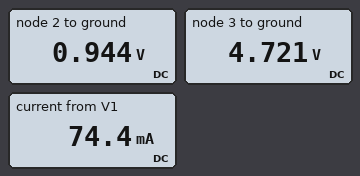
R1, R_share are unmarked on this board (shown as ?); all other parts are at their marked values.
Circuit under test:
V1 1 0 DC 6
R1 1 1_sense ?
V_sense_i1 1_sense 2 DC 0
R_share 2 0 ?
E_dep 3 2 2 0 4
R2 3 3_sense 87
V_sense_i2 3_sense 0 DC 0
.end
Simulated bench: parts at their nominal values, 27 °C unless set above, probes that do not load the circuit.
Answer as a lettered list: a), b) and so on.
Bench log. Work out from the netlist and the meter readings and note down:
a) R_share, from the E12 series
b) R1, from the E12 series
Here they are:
a) 47 Ω
b) 68 Ω
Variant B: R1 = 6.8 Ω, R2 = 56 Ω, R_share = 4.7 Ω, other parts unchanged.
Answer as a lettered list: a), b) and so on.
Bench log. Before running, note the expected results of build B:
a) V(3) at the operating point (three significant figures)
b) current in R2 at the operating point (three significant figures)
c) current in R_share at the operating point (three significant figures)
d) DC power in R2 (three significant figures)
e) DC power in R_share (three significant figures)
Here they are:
a) 9.82 V
b) 175 mA
c) 418 mA
d) 1.72 W
e) 821 mW
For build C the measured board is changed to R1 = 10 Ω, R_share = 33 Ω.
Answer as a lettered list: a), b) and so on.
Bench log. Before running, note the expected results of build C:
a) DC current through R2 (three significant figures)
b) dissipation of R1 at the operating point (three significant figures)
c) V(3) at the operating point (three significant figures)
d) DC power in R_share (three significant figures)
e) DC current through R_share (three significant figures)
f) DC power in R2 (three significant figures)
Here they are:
a) 184 mA
b) 787 mW
c) 16.0 V
d) 309 mW
e) 96.8 mA
f) 2.93 W
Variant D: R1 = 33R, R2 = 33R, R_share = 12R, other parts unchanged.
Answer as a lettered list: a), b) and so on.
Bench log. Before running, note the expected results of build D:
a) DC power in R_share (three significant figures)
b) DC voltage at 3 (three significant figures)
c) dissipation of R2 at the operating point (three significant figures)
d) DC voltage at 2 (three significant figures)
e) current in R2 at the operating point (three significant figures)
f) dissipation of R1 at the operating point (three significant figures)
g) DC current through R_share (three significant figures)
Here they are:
a) 39.2 mW
b) 3.43 V
c) 356 mW
d) 686 mV
e) 104 mA
f) 856 mW
g) 57.1 mA
